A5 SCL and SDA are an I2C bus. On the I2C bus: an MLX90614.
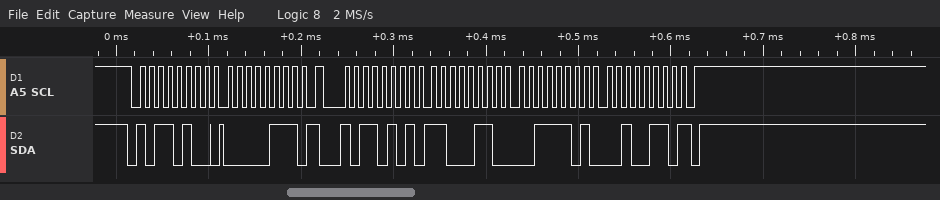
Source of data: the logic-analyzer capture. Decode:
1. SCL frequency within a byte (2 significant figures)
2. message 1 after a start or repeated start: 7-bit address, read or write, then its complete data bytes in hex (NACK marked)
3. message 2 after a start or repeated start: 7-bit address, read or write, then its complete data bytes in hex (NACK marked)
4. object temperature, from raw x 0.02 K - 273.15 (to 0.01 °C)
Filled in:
100 kHz
0x5A write: 07
0x5A read: C6 3D 26 NACK
43.13 °C
